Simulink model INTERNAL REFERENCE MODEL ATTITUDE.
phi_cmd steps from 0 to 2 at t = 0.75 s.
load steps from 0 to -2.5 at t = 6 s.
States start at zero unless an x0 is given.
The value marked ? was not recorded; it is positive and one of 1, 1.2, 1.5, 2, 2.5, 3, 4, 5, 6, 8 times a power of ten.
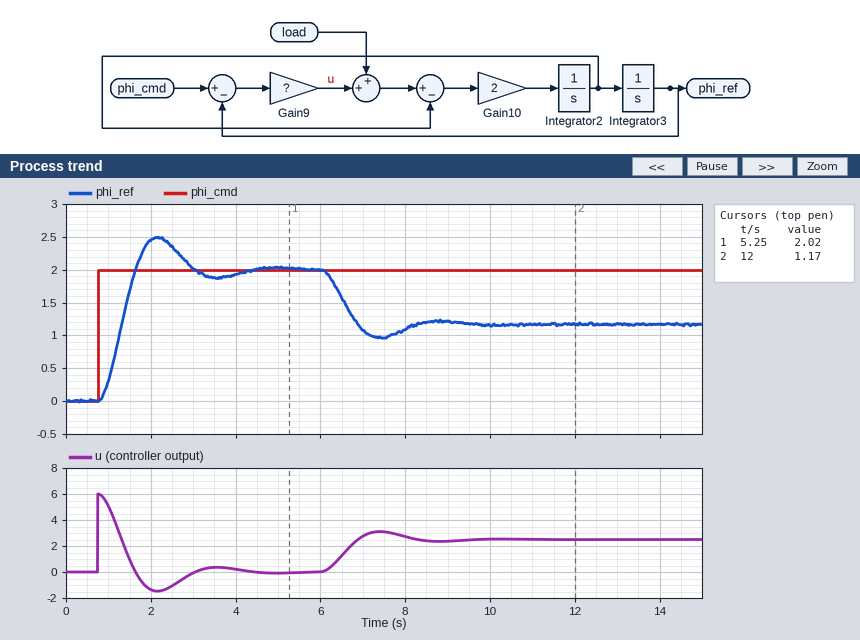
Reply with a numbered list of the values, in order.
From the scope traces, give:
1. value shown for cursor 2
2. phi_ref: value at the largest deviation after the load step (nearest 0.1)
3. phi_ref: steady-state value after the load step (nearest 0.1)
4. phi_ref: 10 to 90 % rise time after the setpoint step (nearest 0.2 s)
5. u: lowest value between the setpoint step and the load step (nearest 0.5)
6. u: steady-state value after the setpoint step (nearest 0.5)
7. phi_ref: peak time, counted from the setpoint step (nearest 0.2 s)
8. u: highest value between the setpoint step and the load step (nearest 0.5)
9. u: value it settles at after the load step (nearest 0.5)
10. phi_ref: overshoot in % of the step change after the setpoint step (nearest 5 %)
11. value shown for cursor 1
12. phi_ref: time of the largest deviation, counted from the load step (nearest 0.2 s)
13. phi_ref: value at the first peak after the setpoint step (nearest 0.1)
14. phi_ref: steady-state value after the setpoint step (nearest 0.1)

1. 1.17
2. 1.0
3. 1.2
4. 0.6 s
5. -1.5
6. 0.0
7. 1.4 s
8. 6.0
9. 2.5
10. 25 %
11. 2.02
12. 1.4 s
13. 2.5
14. 2.0
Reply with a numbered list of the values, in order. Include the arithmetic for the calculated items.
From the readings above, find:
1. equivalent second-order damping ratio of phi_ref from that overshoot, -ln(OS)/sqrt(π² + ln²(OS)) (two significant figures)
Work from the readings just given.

1. ln(0.25) = -1.386; 1.386 / sqrt(9.870 + 1.922) = 0.40
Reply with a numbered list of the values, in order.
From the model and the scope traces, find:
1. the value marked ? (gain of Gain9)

1. 3
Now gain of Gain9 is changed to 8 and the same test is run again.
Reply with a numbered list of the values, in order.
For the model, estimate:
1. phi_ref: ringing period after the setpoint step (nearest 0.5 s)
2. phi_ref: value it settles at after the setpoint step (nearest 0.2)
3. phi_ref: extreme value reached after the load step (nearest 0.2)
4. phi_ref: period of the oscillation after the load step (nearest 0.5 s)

1. 1.5 s
2. 2.0
3. 1.6
4. 1.5 s
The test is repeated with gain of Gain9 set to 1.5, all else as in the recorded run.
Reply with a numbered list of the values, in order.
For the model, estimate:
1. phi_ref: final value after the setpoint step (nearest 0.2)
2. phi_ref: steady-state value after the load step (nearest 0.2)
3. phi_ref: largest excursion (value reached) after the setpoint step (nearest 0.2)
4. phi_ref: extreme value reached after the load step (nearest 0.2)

1. 2.0
2. 0.4
3. 2.2
4. 0.2
